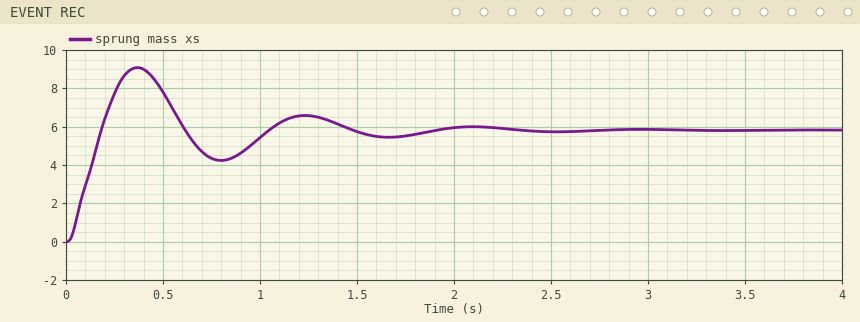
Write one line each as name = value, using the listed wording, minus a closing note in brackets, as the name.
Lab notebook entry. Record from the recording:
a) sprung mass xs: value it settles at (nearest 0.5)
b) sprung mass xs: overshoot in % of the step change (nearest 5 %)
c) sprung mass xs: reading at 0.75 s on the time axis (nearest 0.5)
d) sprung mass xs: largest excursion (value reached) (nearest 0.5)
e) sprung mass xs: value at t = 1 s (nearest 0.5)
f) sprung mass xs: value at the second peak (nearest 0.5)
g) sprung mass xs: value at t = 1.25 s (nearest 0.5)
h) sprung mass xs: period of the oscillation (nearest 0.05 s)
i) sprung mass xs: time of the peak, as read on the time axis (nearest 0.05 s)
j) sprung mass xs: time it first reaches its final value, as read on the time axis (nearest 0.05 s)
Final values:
sprung mass xs: value it settles at = 6.0
sprung mass xs: overshoot in % of the step change = 55 %
sprung mass xs: reading at 0.75 s on the time axis = 4.5
sprung mass xs: largest excursion (value reached) = 9.0
sprung mass xs: value at t = 1 s = 5.5
sprung mass xs: value at the second peak = 6.5
sprung mass xs: value at t = 1.25 s = 6.5
sprung mass xs: period of the oscillation = 0.85 s
sprung mass xs: time of the peak, as read on the time axis = 0.35 s
sprung mass xs: time it first reaches its final value, as read on the time axis = 0.20 s
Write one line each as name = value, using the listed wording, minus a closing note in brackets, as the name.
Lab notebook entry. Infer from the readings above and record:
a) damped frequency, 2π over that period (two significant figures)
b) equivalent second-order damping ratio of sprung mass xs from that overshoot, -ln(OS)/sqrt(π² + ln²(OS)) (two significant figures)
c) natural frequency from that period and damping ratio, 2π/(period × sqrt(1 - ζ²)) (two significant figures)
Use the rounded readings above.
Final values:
damped frequency, 2π over that period = 7.4 rad/s
equivalent second-order damping ratio of sprung mass xs from that overshoot, -ln(OS)/sqrt(π² + ln²(OS)) = 0.19
natural frequency from that period and damping ratio, 2π/(period × sqrt(1 - ζ²)) = 7.5 rad/s
